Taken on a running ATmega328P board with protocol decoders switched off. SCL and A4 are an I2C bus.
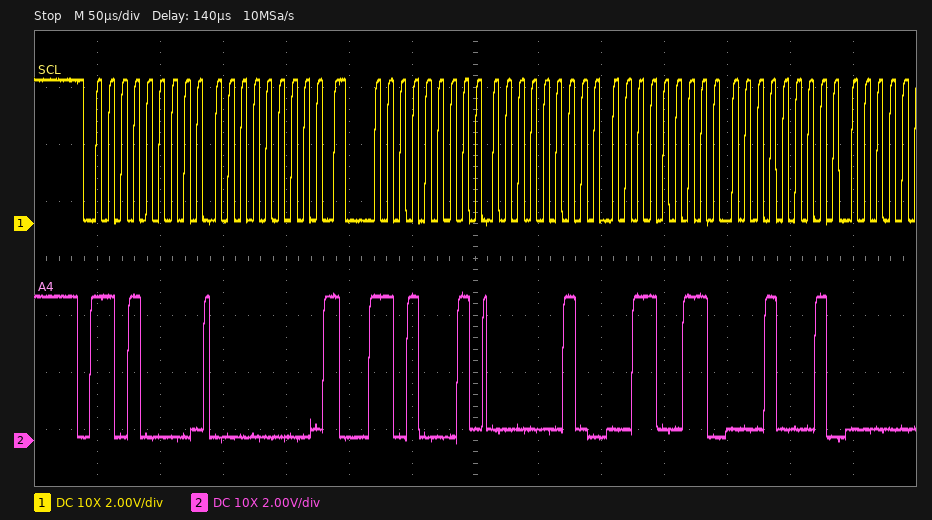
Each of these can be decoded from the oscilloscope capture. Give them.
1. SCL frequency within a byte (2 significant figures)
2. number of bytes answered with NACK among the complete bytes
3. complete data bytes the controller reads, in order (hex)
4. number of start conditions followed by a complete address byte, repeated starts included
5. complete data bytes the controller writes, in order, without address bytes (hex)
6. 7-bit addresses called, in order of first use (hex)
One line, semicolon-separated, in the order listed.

100 kHz; 0; 02 33 11; 2; 00; 0x68
